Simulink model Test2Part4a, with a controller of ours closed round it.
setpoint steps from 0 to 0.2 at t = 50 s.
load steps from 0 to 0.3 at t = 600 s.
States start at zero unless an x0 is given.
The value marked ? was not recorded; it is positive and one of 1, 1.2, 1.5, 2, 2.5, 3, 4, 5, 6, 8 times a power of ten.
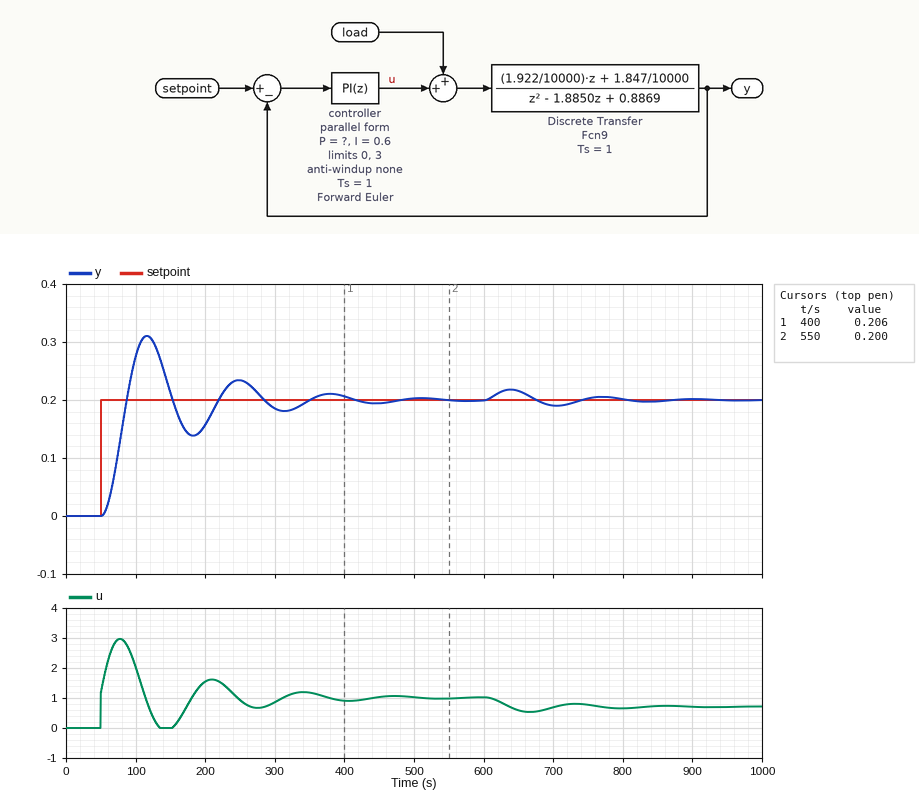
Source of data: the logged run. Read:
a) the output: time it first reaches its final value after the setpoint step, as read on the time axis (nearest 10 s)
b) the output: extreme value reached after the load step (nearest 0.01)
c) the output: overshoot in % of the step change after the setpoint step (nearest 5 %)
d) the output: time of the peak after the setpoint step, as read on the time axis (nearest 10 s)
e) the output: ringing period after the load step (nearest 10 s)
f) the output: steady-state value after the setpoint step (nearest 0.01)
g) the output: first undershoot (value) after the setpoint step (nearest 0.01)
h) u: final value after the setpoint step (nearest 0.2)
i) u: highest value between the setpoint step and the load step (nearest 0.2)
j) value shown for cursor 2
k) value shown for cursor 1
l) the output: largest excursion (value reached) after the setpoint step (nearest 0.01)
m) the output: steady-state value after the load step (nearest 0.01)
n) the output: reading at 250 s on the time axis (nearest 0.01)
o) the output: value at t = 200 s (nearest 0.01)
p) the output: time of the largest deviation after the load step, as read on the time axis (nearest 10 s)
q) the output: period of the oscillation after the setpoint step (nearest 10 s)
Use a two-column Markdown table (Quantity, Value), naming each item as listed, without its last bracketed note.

| Quantity | Value |
|---|---|
| the output: time it first reaches its final value after the setpoint step, as read on the time axis | 90 s |
| the output: extreme value reached after the load step | 0.22 |
| the output: overshoot in % of the step change after the setpoint step | 55 % |
| the output: time of the peak after the setpoint step, as read on the time axis | 120 s |
| the output: ringing period after the load step | 130 s |
| the output: steady-state value after the setpoint step | 0.20 |
| the output: first undershoot (value) after the setpoint step | 0.14 |
| u: final value after the setpoint step | 1.0 |
| u: highest value between the setpoint step and the load step | 3.0 |
| value shown for cursor 2 | 0.200 |
| value shown for cursor 1 | 0.206 |
| the output: largest excursion (value reached) after the setpoint step | 0.31 |
| the output: steady-state value after the load step | 0.20 |
| the output: reading at 250 s on the time axis | 0.23 |
| the output: value at t = 200 s | 0.16 |
| the output: time of the largest deviation after the load step, as read on the time axis | 640 s |
| the output: period of the oscillation after the setpoint step | 130 s |
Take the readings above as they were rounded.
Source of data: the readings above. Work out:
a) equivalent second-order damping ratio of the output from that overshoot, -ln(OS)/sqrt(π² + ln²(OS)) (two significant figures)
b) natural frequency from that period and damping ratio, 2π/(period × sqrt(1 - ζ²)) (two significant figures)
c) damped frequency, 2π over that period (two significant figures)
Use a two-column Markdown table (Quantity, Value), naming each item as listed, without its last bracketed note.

| Quantity | Value |
|---|---|
| equivalent second-order damping ratio of the output from that overshoot, -ln(OS)/sqrt(π² + ln²(OS)) | 0.19 |
| natural frequency from that period and damping ratio, 2π/(period × sqrt(1 - ζ²)) | 0.049 rad/s |
| damped frequency, 2π over that period | 0.048 rad/s |
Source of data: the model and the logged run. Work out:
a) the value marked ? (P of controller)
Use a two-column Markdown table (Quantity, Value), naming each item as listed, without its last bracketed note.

| Quantity | Value |
|---|---|
| the value marked ? | 6 |
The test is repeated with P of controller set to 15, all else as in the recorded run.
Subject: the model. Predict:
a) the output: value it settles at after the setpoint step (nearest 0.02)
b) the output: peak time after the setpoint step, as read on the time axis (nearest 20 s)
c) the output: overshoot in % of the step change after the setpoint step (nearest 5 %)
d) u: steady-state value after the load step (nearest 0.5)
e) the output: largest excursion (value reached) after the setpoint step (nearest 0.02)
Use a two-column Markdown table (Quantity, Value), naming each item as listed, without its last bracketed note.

| Quantity | Value |
|---|---|
| the output: value it settles at after the setpoint step | 0.20 |
| the output: peak time after the setpoint step, as read on the time axis | 100 s |
| the output: overshoot in % of the step change after the setpoint step | 30 % |
| u: steady-state value after the load step | 0.5 |
| the output: largest excursion (value reached) after the setpoint step | 0.26 |
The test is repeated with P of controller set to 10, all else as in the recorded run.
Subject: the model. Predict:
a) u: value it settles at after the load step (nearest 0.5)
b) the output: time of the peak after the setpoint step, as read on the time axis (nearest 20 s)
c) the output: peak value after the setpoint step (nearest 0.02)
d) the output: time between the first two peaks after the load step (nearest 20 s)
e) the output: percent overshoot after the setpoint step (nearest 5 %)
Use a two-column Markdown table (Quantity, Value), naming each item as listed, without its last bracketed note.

| Quantity | Value |
|---|---|
| u: value it settles at after the load step | 0.5 |
| the output: time of the peak after the setpoint step, as read on the time axis | 100 s |
| the output: peak value after the setpoint step | 0.28 |
| the output: time between the first two peaks after the load step | 120 s |
| the output: percent overshoot after the setpoint step | 40 % |
